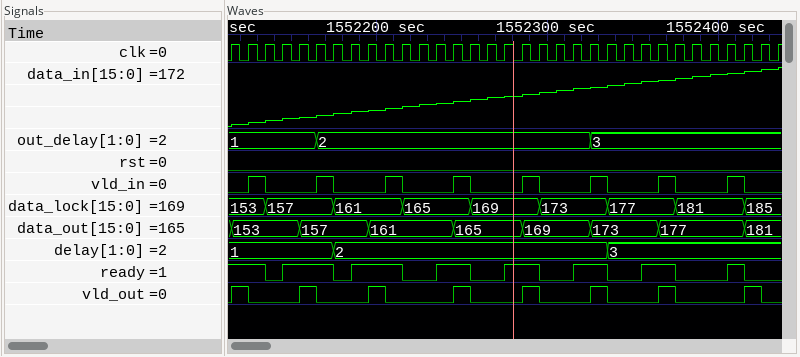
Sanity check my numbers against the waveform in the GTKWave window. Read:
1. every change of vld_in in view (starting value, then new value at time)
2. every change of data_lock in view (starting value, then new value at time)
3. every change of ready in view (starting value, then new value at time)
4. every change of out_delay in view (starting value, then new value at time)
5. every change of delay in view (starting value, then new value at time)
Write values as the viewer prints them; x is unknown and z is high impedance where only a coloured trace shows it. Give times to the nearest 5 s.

0, 1 at 1552125 s, 0 at 1552135 s, 1 at 1552165 s, 0 at 1552175 s, 1 at 1552205 s, 0 at 1552215 s, 1 at 1552245 s, 0 at 1552255 s, 1 at 1552285 s, 0 at 1552295 s, 1 at 1552325 s, 0 at 1552335 s, 1 at 1552365 s, 0 at 1552375 s, 1 at 1552405 s, 0 at 1552415 s
153, 157 at 1552135 s, 161 at 1552175 s, 165 at 1552215 s, 169 at 1552255 s, 173 at 1552295 s, 177 at 1552335 s, 181 at 1552375 s, 185 at 1552415 s
1, 0 at 1552135 s, 1 at 1552145 s, 0 at 1552175 s, 1 at 1552185 s, 0 at 1552215 s, 1 at 1552235 s, 0 at 1552255 s, 1 at 1552275 s, 0 at 1552295 s, 1 at 1552315 s, 0 at 1552335 s, 1 at 1552355 s, 0 at 1552375 s, 1 at 1552405 s, 0 at 1552415 s
1, 2 at 1552165 s, 3 at 1552325 s
1, 2 at 1552175 s, 3 at 1552335 s
